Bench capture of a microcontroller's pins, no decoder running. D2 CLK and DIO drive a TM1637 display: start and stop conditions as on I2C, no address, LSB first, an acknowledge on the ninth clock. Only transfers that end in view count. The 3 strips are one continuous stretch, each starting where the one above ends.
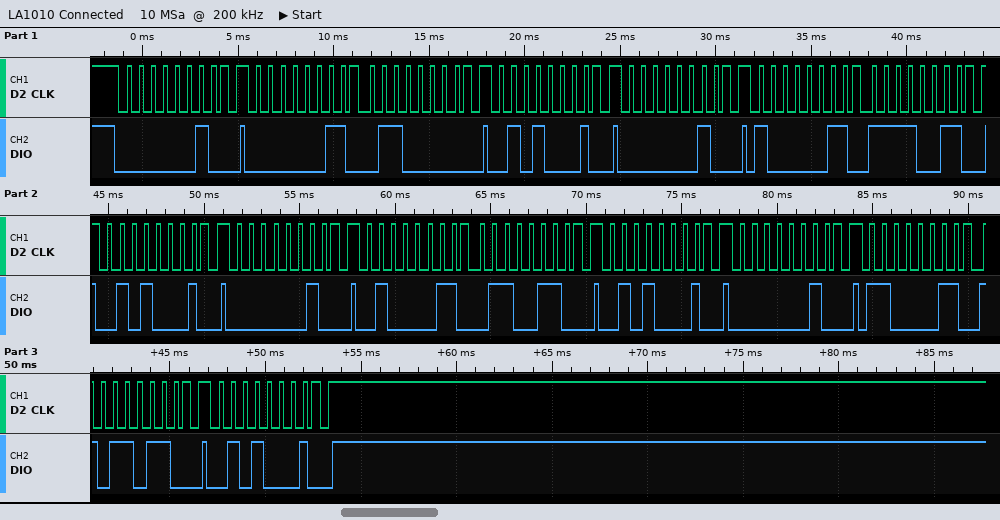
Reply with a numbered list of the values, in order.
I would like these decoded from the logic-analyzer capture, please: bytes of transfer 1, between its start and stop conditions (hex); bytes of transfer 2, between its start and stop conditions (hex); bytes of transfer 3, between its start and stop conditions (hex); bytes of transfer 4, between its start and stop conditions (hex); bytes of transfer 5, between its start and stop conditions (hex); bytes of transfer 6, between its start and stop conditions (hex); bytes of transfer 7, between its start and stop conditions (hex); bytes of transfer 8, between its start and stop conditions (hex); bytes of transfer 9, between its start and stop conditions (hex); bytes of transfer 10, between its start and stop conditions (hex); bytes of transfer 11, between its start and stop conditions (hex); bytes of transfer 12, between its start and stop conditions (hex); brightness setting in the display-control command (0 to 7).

1. 40
2. C0 06
3. 8A
4. 40
5. C1 CF
6. 8A
7. 40
8. C2 66
9. 8A
10. 40
11. C3 6D
12. 8A
13. 2
